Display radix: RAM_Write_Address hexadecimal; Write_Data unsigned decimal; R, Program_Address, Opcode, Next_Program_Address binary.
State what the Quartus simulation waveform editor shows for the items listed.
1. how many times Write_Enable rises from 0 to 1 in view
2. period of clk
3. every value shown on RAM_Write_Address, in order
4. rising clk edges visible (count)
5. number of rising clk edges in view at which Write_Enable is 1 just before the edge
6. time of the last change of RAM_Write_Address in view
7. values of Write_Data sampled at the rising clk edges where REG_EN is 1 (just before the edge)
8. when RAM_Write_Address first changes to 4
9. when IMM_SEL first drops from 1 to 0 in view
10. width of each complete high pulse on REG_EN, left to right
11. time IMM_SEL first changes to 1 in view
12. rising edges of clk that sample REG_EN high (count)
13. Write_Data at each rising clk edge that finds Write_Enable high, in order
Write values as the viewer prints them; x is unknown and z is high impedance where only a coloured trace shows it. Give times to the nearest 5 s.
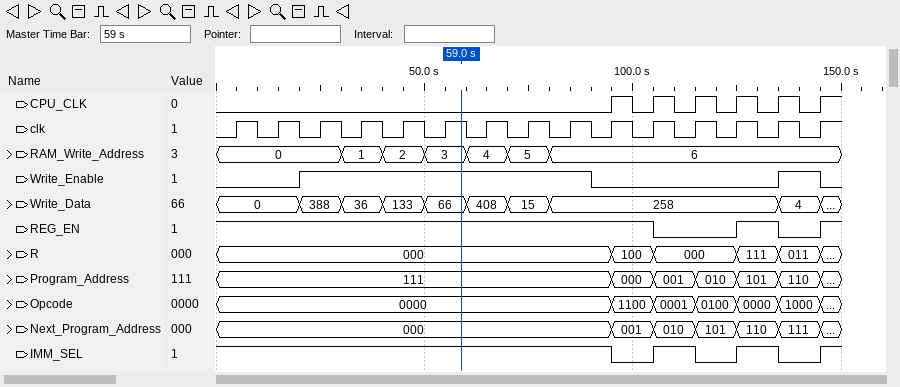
2
10 s
0, 1, 2, 3, 4, 5, 6
15
8
80 s
0, 0, 388, 36, 133, 66, 408, 15, 258, 258, 258, 258
60 s
95 s
10 s
105 s
12
388, 36, 133, 66, 408, 15, 258, 4
